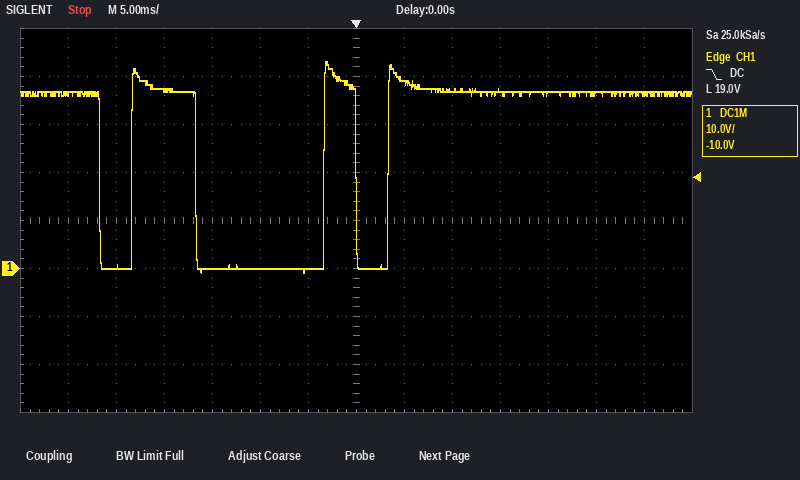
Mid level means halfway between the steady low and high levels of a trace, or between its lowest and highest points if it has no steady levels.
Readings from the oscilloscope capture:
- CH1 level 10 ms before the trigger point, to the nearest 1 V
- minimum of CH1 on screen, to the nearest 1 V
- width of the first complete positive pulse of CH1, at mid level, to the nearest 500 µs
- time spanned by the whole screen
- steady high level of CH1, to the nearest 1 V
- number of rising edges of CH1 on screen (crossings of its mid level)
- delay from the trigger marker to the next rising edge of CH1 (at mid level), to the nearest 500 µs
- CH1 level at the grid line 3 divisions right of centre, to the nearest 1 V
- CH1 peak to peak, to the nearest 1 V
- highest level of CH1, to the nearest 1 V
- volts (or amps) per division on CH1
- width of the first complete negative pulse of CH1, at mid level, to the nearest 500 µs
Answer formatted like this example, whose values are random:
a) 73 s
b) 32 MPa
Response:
a) 0 V
b) -1 V
c) 6.5 ms
d) 70 ms
e) 37 V
f) 3
g) 3.5 ms
h) 37 V
i) 44 V
j) 43 V
k) 10 V
l) 3.5 ms
